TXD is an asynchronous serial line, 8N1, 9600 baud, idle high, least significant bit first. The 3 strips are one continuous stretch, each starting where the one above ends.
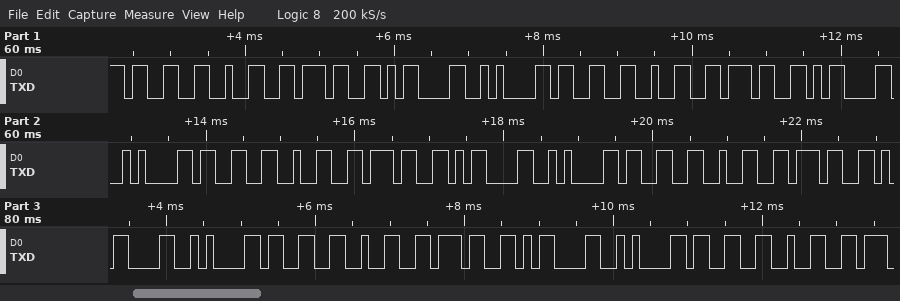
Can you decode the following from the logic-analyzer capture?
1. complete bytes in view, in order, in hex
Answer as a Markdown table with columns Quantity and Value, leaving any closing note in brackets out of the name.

| Quantity | Value |
|---|---|
| complete bytes in view, in order, in hex | 33 32 37 0D 0A 33 32 37 0D 0A 33 32 37 0D 0A 33 32 37 0D 0A 33 32 37 0D 0A 33 32 |
